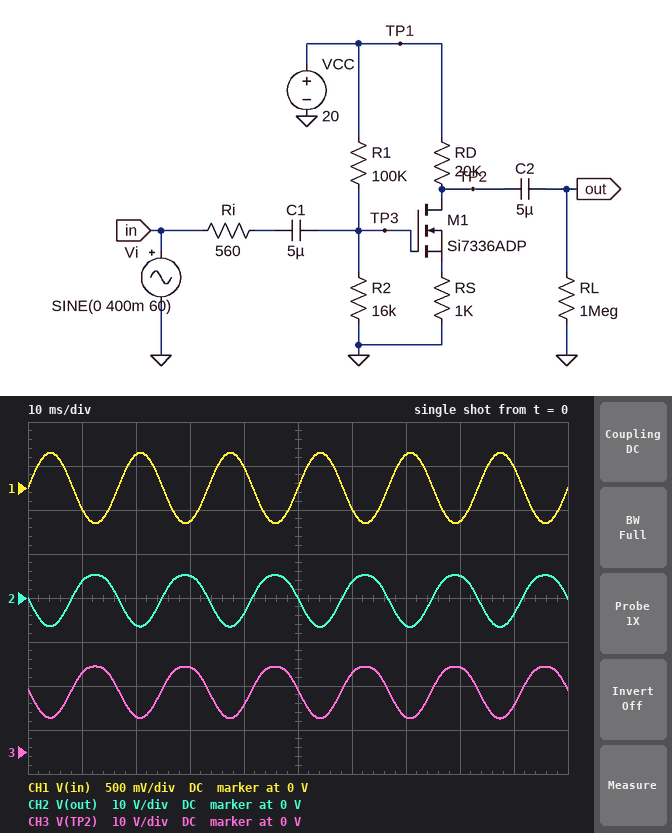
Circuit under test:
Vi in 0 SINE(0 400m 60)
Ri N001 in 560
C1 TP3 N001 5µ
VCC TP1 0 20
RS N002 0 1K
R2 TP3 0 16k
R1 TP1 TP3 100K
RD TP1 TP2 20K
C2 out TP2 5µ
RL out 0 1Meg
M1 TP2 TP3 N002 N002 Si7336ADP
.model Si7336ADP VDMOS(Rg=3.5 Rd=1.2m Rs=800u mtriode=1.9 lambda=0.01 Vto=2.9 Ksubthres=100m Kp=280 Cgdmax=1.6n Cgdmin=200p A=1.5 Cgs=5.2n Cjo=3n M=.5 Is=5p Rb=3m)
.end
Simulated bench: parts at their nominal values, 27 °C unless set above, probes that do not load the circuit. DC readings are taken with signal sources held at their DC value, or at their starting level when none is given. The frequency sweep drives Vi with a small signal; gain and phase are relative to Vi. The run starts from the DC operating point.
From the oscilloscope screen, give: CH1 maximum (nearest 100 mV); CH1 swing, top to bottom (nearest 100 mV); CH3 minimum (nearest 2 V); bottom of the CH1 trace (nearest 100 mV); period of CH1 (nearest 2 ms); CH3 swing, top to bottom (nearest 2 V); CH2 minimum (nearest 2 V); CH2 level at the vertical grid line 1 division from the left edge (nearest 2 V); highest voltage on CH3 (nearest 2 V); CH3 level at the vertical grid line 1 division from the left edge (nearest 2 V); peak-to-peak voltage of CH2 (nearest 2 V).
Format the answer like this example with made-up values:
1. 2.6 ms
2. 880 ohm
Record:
1. 400 mV
2. 800 mV
3. 8 V
4. -400 mV
5. 16 ms
6. 12 V
7. -6 V
8. 4 V
9. 20 V
10. 18 V
11. 12 V
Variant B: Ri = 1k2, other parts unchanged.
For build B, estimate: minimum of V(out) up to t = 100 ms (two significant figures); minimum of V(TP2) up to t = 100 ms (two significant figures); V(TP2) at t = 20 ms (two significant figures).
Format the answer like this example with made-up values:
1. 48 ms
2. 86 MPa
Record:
1. -6.3 V
2. 7.9 V
3. 8.3 V
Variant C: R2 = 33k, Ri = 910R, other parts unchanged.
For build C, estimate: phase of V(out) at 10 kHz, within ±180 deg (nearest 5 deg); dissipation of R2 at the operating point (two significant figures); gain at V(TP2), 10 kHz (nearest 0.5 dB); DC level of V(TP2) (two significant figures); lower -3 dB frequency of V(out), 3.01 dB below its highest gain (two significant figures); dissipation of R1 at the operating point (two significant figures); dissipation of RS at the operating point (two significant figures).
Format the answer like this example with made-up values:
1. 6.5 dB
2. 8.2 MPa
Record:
1. 50 deg
2. 750 µW
3. -10.0 dB
4. 950 mV
5. 13 kHz
6. 2.3 mW
7. 910 µW
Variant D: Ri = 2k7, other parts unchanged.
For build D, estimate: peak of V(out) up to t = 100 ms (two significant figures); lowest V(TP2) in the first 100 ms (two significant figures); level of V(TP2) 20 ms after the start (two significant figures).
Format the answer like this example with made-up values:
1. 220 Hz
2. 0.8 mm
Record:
1. 4.8 V
2. 8.5 V
3. 8.8 V
